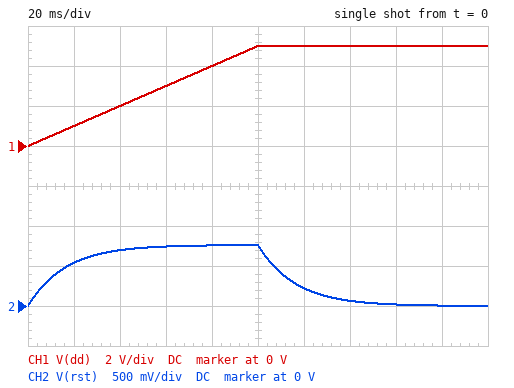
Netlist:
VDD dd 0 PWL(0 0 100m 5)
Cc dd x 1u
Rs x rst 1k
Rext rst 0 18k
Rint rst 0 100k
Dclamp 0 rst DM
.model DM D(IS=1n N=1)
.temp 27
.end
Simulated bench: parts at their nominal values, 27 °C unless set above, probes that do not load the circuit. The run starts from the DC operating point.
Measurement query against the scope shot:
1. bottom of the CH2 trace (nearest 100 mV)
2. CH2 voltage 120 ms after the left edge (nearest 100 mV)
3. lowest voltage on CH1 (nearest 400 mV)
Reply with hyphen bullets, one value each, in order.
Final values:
- 0 V
- 200 mV
- 0 V
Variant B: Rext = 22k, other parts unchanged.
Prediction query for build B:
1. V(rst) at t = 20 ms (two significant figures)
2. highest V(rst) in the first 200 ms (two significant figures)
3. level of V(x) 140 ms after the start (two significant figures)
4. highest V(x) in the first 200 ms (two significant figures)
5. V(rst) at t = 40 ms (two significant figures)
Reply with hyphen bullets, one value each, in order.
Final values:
- 590 mV
- 900 mV
- 120 mV
- 950 mV
- 790 mV
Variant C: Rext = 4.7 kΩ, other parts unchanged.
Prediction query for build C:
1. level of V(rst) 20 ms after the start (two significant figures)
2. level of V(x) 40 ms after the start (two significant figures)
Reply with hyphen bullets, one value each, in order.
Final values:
- 220 mV
- 270 mV
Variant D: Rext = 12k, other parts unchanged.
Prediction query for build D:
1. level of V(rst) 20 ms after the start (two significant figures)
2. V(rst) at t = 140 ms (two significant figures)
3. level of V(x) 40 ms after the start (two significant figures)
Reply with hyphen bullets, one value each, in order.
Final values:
- 440 mV
- 18 mV
- 570 mV
